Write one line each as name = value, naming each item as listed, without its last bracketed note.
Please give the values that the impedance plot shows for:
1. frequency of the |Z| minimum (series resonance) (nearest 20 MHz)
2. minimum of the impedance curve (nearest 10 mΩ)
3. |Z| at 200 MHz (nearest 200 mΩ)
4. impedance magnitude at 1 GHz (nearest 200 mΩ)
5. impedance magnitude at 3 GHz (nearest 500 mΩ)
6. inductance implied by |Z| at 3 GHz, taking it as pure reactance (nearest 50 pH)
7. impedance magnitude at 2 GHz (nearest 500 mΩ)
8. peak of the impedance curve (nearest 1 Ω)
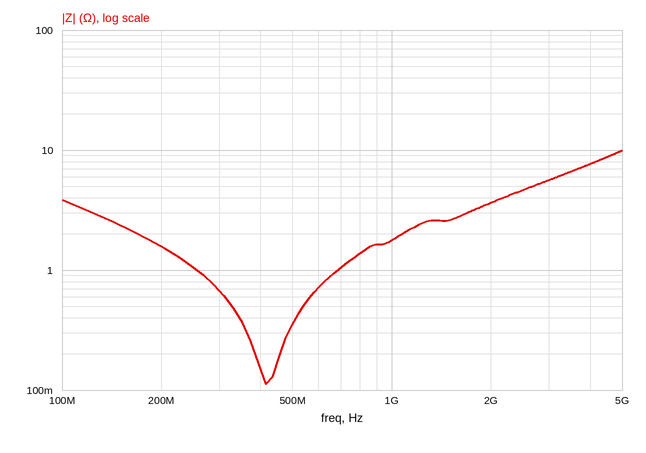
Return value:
frequency of the |Z| minimum (series resonance) = 420 MHz
minimum of the impedance curve = 110 mΩ
|Z| at 200 MHz = 1.6 Ω
impedance magnitude at 1 GHz = 1.8 Ω
impedance magnitude at 3 GHz = 5.5 Ω
inductance implied by |Z| at 3 GHz, taking it as pure reactance = 300 pH
impedance magnitude at 2 GHz = 3.5 Ω
peak of the impedance curve = 10 Ω
